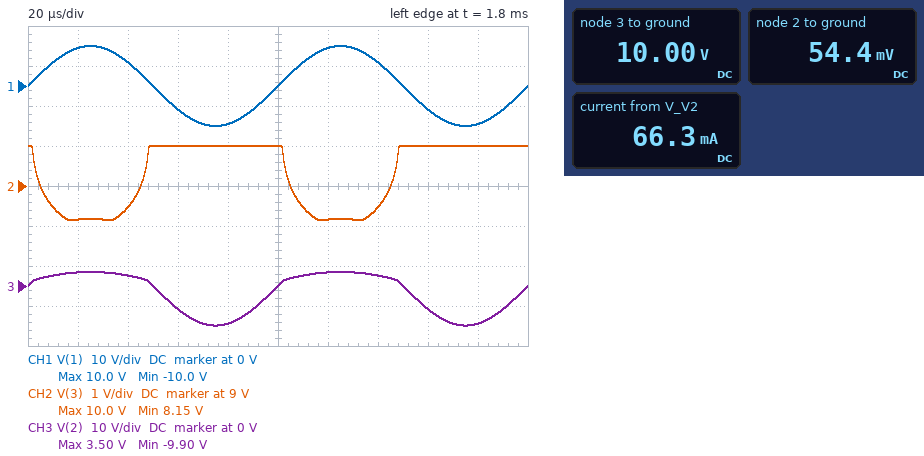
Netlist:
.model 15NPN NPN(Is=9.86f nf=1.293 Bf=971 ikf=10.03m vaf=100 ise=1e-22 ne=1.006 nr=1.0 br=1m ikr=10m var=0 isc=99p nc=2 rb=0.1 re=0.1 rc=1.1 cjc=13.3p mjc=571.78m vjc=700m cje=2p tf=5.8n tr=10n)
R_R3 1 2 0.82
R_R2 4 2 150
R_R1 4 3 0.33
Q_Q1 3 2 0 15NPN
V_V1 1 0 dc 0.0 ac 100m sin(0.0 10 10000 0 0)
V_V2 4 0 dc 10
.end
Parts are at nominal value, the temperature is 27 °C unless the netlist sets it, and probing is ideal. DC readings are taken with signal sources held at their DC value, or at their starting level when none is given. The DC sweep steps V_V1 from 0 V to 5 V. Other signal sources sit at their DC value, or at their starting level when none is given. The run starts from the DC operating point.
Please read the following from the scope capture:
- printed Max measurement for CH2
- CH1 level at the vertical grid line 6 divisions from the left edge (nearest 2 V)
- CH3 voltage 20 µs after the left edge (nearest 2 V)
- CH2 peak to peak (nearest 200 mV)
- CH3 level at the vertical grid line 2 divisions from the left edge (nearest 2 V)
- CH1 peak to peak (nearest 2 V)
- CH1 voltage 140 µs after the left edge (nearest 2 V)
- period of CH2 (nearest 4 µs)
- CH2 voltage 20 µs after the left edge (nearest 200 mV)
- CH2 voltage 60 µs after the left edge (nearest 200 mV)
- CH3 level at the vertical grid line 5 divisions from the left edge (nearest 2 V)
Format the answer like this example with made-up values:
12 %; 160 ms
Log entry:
10.0 V; 10 V; 4 V; 1.8 V; 2 V; 20 V; 6 V; 100 µs; 8.2 V; 10.0 V; 0 V
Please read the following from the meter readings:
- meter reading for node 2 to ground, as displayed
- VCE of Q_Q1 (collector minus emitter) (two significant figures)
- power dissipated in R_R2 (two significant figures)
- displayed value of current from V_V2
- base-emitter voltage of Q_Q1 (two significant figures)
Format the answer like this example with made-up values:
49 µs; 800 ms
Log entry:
54.4 mV; 10 V; 660 mW; 66.3 mA; 54 mV
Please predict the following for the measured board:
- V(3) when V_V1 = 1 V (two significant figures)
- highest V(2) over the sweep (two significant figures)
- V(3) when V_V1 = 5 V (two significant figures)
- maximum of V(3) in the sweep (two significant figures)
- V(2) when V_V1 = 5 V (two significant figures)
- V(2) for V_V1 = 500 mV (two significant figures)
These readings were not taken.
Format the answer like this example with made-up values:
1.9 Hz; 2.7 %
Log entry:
10 V; 2.4 V; 8.6 V; 10 V; 2.4 V; 550 mV
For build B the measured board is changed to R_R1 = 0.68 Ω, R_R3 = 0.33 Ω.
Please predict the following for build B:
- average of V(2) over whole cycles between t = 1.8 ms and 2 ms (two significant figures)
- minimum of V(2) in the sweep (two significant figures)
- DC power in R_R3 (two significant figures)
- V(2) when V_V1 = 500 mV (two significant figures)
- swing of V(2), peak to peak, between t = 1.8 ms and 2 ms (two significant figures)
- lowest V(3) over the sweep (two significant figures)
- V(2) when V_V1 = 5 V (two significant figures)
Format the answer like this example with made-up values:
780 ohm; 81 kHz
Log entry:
-1.4 V; 22 mV; 1.5 mW; 520 mV; 15 V; 6.8 V; 3.0 V
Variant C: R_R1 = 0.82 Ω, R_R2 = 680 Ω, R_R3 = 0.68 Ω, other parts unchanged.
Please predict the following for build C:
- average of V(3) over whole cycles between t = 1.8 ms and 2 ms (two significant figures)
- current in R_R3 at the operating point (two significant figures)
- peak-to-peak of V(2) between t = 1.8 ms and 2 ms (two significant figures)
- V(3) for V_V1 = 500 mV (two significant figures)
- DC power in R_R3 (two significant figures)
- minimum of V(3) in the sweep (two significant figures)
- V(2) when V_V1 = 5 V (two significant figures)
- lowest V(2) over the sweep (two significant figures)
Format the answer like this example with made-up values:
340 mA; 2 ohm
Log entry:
8.5 V; 15 mA; 14 V; 10 V; 150 µW; 6.4 V; 2.5 V; 10 mV
